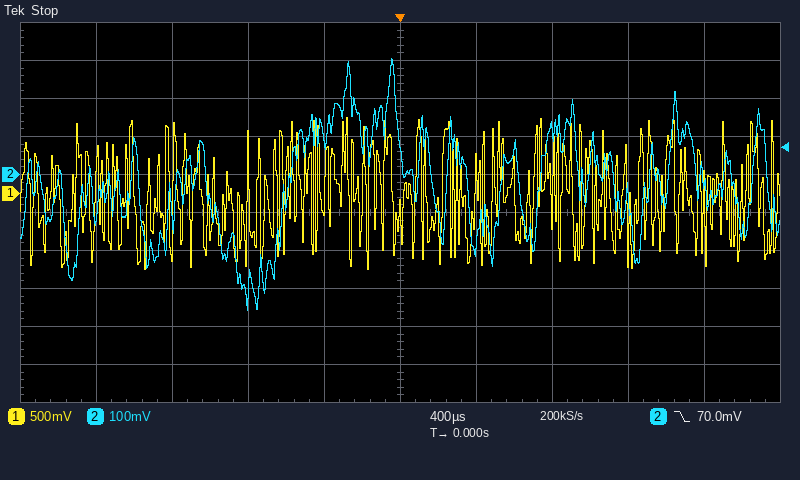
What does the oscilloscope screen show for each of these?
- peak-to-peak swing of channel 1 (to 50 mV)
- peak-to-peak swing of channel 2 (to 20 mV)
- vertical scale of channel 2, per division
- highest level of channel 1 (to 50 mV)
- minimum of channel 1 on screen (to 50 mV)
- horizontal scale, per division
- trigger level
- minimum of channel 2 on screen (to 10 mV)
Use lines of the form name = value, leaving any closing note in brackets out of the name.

peak-to-peak swing of channel 1 = 2.00 V
peak-to-peak swing of channel 2 = 660 mV
vertical scale of channel 2, per division = 100 mV
highest level of channel 1 = 1.00 V
minimum of channel 1 on screen = -1.00 V
horizontal scale, per division = 400 µs
trigger level = 70.0 mV
minimum of channel 2 on screen = -360 mV
